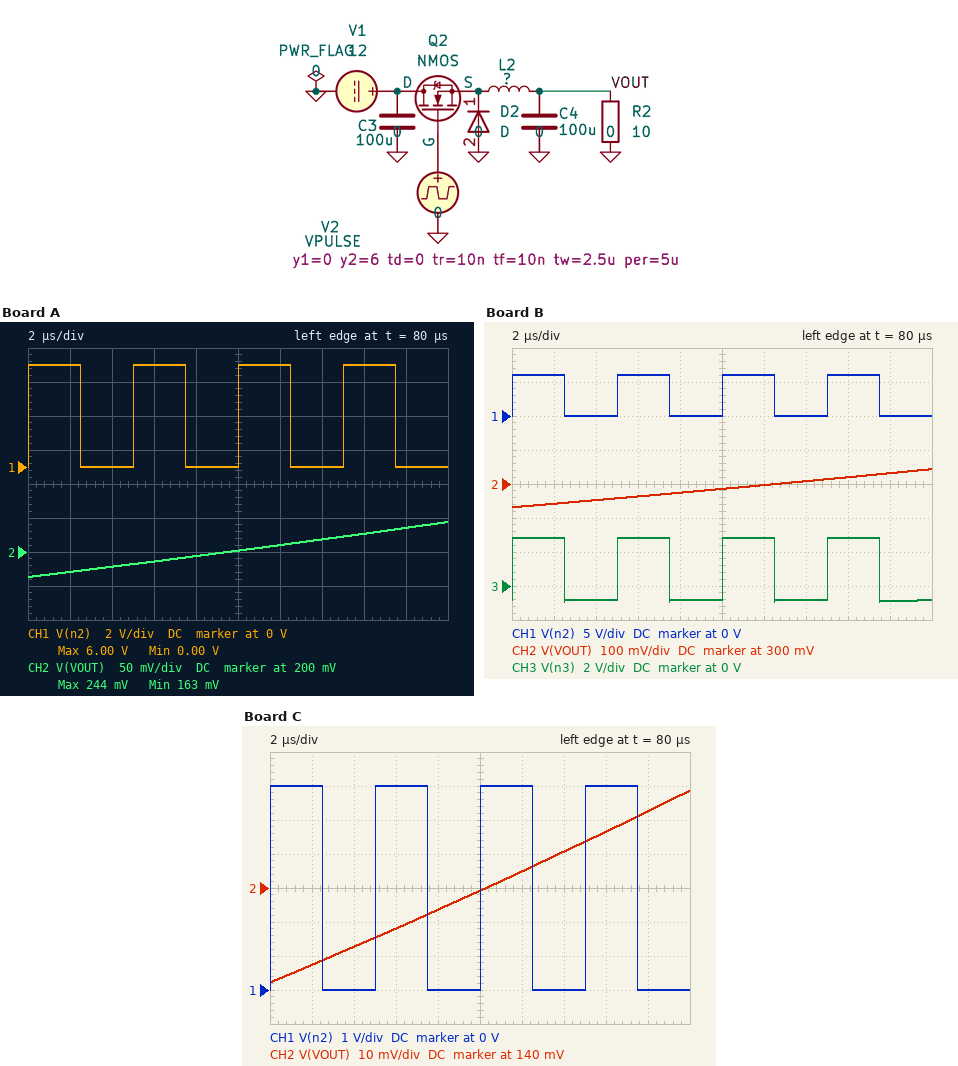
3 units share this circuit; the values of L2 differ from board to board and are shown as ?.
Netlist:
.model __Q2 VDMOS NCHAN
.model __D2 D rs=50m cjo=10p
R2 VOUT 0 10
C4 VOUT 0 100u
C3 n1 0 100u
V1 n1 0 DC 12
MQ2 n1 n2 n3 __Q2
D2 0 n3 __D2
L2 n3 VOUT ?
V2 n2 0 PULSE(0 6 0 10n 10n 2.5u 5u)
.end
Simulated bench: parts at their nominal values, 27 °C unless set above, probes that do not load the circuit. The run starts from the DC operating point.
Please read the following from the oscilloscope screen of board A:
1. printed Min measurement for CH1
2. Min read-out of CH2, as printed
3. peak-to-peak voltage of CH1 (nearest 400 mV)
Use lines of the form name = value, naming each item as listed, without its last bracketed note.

printed Min measurement for CH1 = 0.00 V
Min read-out of CH2, as printed = 163 mV
peak-to-peak voltage of CH1 = 6.0 V
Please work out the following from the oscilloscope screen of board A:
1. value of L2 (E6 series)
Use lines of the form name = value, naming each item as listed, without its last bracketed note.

value of L2 = 220 µH
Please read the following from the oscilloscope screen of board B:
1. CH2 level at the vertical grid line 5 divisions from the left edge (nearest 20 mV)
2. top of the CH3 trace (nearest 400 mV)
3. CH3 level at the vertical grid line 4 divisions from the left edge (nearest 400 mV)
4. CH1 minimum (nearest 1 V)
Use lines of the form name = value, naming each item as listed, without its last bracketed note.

CH2 level at the vertical grid line 5 divisions from the left edge = 280 mV
top of the CH3 trace = 2.8 V
CH3 level at the vertical grid line 4 divisions from the left edge = -800 mV
CH1 minimum = 0 V
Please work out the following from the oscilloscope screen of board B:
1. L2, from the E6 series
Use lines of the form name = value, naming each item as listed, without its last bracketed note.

L2, from the E6 series = 150 µH
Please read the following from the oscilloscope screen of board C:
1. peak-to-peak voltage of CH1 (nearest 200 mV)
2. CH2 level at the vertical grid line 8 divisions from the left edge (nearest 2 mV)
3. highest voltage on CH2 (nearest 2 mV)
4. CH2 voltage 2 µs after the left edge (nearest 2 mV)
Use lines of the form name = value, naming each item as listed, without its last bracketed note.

peak-to-peak voltage of CH1 = 6.0 V
CH2 level at the vertical grid line 8 divisions from the left edge = 156 mV
highest voltage on CH2 = 168 mV
CH2 voltage 2 µs after the left edge = 118 mV
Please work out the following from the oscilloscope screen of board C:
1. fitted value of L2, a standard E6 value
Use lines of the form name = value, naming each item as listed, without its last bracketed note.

fitted value of L2, a standard E6 value = 330 µH
